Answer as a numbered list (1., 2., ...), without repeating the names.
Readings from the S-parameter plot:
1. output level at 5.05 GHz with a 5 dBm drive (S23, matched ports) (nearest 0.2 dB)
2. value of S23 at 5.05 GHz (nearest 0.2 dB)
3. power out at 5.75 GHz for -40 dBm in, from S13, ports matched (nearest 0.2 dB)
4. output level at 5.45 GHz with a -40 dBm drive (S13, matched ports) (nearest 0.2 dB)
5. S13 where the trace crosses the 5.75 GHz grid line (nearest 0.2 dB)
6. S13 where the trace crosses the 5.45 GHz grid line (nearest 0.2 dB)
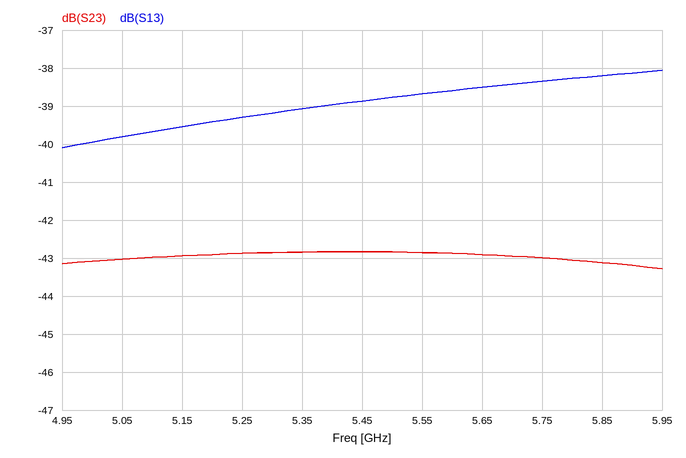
1. -38.0 dBm
2. -43.0 dB
3. -78.4 dBm
4. -78.8 dBm
5. -38.4 dB
6. -38.8 dB
